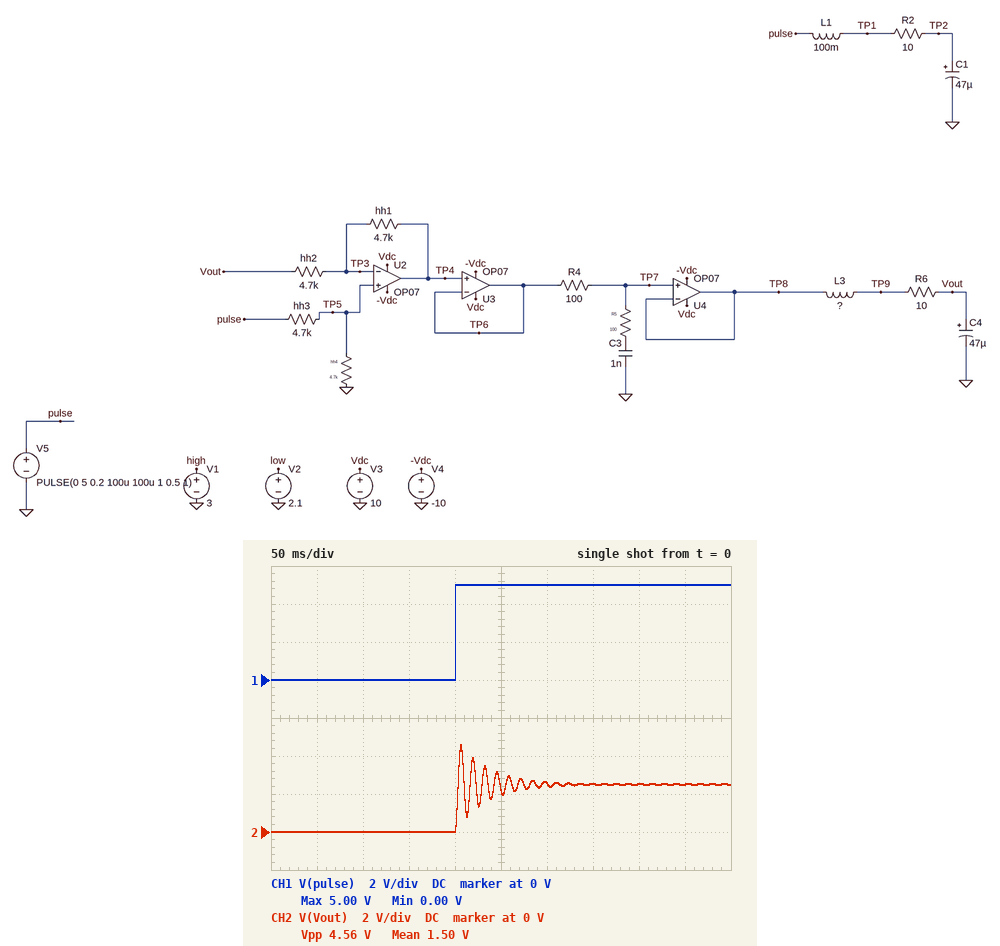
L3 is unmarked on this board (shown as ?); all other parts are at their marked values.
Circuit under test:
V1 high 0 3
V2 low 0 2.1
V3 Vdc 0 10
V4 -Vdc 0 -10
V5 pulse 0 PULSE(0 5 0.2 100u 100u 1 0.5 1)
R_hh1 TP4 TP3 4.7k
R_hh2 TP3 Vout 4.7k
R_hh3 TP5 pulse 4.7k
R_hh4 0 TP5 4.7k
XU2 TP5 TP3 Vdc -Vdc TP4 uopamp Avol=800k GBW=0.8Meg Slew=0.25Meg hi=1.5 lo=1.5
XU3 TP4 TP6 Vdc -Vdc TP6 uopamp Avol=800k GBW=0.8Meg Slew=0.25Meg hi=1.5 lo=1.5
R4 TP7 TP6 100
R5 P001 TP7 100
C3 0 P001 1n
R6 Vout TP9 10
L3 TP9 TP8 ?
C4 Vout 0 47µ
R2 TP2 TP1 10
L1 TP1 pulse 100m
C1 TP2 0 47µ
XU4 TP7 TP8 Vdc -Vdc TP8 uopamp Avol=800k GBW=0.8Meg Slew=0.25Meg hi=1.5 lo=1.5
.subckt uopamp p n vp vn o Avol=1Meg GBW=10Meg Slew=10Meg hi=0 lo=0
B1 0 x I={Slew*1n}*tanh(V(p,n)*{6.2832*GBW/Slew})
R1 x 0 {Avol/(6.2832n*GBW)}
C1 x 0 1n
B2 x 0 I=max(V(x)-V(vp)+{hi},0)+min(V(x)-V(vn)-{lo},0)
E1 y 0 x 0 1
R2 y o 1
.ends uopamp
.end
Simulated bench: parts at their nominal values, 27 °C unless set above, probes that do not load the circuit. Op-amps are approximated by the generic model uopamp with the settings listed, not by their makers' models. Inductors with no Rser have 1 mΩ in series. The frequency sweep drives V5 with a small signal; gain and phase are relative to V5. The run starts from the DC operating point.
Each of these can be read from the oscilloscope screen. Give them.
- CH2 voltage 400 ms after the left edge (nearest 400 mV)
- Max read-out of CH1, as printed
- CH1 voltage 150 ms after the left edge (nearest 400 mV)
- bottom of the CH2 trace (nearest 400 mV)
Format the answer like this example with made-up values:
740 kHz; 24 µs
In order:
2.4 V; 5.00 V; 0 V; 0 V
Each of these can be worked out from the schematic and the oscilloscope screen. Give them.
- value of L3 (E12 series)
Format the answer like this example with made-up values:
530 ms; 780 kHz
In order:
180 mH
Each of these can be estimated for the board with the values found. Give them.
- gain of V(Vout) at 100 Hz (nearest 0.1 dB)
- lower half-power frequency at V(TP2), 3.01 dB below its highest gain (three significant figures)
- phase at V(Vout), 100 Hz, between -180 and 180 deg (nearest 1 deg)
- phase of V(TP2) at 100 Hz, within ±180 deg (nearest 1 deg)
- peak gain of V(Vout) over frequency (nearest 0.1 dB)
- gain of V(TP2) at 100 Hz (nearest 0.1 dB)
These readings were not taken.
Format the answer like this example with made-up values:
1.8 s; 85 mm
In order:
-2.8 dB; 64.0 Hz; -166 deg; -161 deg; 12.2 dB; 0.9 dB
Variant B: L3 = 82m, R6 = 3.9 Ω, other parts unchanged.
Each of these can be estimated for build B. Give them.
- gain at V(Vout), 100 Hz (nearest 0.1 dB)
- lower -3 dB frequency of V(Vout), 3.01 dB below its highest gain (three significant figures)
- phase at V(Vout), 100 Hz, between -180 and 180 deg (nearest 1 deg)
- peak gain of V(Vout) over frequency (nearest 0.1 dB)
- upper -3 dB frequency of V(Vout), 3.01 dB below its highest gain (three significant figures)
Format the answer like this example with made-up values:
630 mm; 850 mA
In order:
6.1 dB; 110 Hz; -14 deg; 16.8 dB; 119 Hz
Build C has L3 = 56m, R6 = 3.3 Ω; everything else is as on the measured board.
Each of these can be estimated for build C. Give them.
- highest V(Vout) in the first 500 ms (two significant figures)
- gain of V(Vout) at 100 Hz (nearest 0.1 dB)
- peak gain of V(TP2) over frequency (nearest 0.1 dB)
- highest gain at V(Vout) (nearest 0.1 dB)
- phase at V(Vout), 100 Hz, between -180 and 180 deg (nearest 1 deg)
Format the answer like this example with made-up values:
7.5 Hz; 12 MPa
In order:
4.7 V; 0.3 dB; 13.3 dB; 16.8 dB; -6 deg
